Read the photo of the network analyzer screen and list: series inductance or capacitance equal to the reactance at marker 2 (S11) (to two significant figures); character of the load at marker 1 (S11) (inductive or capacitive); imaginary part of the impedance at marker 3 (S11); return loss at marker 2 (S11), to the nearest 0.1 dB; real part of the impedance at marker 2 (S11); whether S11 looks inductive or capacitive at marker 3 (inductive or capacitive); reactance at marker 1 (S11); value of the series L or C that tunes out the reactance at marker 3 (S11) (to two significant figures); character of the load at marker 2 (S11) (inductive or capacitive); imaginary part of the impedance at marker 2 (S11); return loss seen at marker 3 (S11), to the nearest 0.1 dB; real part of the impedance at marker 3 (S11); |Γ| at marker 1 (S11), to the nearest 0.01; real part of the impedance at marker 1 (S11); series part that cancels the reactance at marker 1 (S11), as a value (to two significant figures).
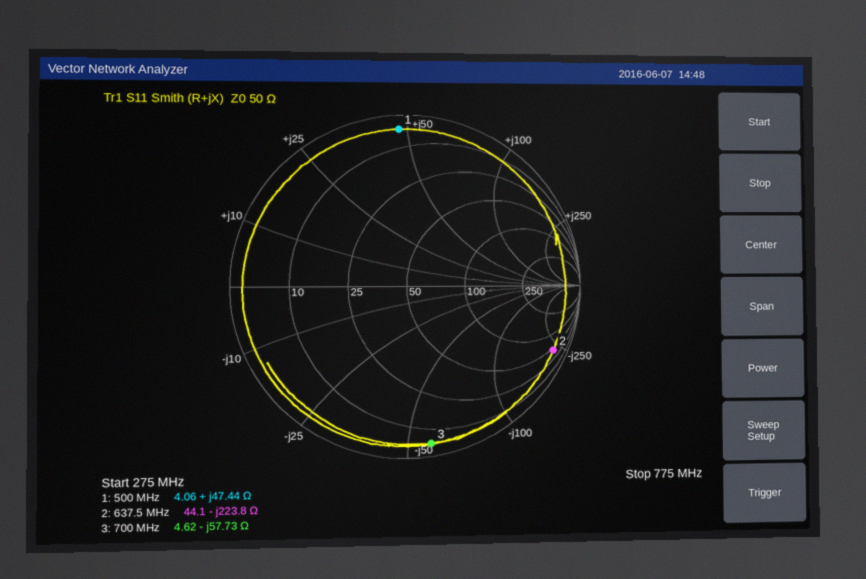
1.1 pF
inductive
-57.73 Ω
0.7 dB
44.1 Ω
capacitive
+47.44 Ω
13 nH
capacitive
-223.8 Ω
0.7 dB
4.62 Ω
0.92
4.06 Ω
6.7 pF
